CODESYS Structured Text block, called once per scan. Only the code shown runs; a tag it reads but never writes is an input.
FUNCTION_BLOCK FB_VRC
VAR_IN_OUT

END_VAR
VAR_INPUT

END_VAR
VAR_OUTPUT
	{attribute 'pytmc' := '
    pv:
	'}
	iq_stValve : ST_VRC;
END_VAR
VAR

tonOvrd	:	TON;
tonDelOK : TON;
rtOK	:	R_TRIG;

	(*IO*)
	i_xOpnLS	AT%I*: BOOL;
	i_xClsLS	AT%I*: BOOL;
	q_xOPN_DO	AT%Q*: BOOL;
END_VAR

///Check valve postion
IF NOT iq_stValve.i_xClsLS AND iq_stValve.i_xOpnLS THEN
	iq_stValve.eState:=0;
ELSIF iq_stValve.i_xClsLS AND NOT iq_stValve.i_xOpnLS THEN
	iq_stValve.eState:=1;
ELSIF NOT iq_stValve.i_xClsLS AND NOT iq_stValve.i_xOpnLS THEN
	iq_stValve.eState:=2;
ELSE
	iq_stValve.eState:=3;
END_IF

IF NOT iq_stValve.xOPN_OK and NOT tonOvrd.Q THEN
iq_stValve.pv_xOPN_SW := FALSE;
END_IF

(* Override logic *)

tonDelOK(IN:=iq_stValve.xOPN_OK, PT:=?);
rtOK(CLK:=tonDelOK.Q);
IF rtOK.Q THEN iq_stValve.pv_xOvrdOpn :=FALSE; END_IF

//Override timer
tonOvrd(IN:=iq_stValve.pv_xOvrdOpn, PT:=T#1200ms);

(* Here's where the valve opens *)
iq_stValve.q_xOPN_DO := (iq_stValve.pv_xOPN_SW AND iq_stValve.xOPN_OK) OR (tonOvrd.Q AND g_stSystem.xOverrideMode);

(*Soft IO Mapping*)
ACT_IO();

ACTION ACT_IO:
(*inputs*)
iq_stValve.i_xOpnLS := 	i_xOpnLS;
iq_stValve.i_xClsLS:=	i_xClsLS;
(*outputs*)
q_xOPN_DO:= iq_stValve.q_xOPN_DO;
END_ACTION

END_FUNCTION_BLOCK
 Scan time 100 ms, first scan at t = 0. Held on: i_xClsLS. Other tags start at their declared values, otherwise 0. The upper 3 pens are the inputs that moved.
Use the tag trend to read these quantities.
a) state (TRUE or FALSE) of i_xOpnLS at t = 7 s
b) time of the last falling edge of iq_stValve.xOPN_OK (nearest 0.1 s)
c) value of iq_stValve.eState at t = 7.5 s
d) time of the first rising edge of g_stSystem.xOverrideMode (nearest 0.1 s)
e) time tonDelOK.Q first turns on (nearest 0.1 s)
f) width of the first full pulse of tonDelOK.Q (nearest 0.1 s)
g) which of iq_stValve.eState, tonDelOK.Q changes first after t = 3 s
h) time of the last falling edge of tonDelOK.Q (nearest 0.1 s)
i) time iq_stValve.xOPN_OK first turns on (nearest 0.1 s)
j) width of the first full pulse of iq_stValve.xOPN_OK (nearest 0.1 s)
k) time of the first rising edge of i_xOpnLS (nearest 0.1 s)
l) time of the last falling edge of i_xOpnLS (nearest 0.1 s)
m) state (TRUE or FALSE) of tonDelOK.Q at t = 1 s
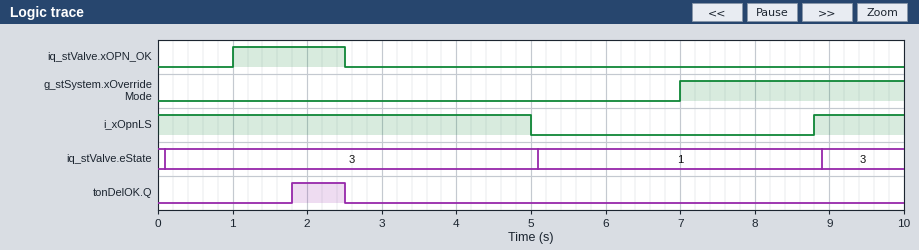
FALSE
2.5 s
1
7.0 s
1.8 s
0.7 s
iq_stValve.eState
2.5 s
1.0 s
1.5 s
8.8 s
5.0 s
FALSE
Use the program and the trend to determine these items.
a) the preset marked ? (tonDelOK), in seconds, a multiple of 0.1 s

0.8 s
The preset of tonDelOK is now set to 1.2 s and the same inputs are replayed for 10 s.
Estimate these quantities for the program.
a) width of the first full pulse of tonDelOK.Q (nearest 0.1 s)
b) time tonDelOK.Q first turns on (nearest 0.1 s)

0.3 s
2.2 s
